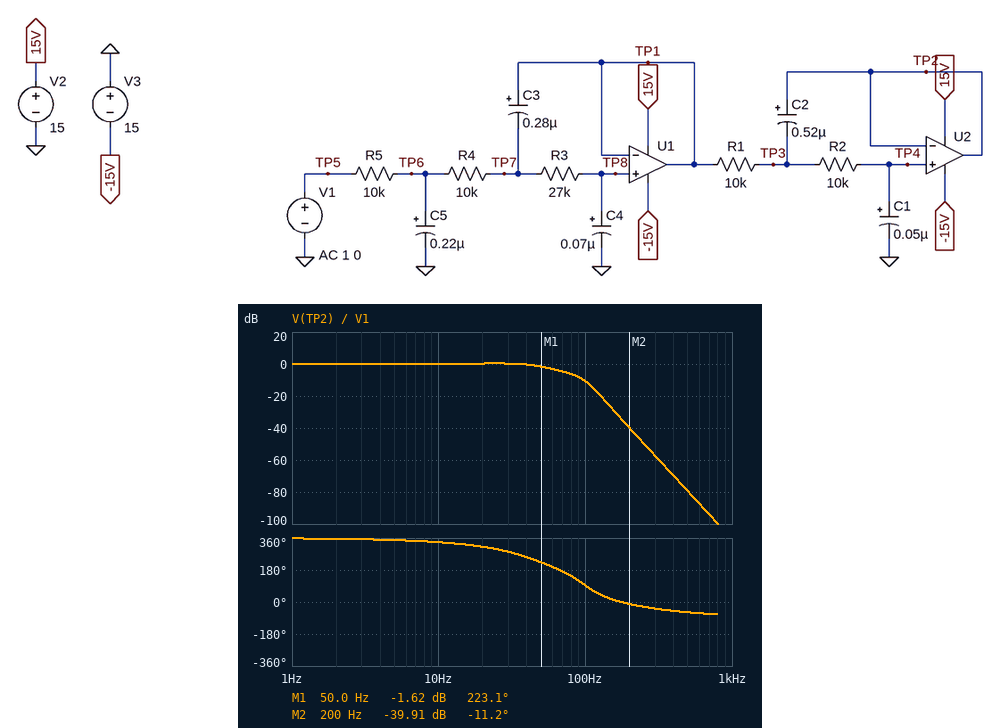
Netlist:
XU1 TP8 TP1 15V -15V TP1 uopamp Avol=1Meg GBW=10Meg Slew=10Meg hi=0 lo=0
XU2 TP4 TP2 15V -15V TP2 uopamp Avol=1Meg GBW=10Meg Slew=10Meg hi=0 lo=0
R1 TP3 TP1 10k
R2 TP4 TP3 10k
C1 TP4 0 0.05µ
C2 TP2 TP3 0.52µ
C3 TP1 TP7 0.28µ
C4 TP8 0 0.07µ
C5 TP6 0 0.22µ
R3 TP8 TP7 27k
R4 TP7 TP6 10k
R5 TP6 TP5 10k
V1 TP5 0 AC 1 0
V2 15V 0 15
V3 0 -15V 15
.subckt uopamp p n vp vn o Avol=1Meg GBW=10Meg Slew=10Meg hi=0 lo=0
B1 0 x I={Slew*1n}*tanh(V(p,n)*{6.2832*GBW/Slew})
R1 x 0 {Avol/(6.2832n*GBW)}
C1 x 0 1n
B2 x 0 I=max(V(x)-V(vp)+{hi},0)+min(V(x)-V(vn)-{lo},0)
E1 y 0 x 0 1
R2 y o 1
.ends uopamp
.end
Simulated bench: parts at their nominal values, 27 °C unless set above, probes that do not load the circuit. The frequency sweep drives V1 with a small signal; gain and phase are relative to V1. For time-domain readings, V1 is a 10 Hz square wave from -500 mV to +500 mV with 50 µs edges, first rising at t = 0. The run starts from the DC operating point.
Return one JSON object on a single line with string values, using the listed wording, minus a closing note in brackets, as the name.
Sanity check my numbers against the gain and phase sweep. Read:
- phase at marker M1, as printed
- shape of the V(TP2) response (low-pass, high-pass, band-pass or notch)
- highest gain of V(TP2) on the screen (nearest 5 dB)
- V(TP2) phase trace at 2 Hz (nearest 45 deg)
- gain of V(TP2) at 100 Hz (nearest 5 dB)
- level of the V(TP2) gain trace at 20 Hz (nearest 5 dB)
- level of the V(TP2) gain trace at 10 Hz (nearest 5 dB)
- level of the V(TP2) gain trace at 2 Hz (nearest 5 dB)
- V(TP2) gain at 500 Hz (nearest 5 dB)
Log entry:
{"phase at marker M1, as printed": "223.1 deg", "shape of the V(TP2) response": "low-pass", "highest gain of V(TP2) on the screen": "0 dB", "V(TP2) phase trace at 2 Hz": "360 deg", "gain of V(TP2) at 100 Hz": "-10 dB", "level of the V(TP2) gain trace at 20 Hz": "0 dB", "level of the V(TP2) gain trace at 10 Hz": "0 dB", "level of the V(TP2) gain trace at 2 Hz": "0 dB", "V(TP2) gain at 500 Hz": "-80 dB"}
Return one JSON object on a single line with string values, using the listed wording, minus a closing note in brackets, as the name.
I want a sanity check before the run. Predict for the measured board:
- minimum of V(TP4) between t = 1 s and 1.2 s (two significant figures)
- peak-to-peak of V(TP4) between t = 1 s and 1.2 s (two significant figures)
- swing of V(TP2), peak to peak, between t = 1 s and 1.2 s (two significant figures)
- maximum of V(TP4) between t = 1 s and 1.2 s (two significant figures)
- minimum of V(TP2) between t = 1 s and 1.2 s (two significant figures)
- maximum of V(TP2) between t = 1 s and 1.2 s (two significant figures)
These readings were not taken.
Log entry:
{"minimum of V(TP4) between t = 1 s and 1.2 s": "-580 mV", "peak-to-peak of V(TP4) between t = 1 s and 1.2 s": "1.2 V", "swing of V(TP2), peak to peak, between t = 1 s and 1.2 s": "1.2 V", "maximum of V(TP4) between t = 1 s and 1.2 s": "580 mV", "minimum of V(TP2) between t = 1 s and 1.2 s": "-580 mV", "maximum of V(TP2) between t = 1 s and 1.2 s": "580 mV"}
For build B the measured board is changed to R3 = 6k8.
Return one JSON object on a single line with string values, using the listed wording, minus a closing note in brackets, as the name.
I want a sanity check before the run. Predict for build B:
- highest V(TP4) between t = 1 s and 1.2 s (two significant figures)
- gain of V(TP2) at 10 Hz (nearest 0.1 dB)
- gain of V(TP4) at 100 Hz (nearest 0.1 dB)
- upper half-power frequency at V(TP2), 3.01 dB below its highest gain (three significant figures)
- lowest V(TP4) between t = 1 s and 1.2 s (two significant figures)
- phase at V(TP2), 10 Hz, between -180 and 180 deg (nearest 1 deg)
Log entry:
{"highest V(TP4) between t = 1 s and 1.2 s": "610 mV", "gain of V(TP2) at 10 Hz": "0 dB", "gain of V(TP4) at 100 Hz": "-2.5 dB", "upper half-power frequency at V(TP2), 3.01 dB below its highest gain": "102 Hz", "lowest V(TP4) between t = 1 s and 1.2 s": "-610 mV", "phase at V(TP2), 10 Hz, between -180 and 180 deg": "-18 deg"}
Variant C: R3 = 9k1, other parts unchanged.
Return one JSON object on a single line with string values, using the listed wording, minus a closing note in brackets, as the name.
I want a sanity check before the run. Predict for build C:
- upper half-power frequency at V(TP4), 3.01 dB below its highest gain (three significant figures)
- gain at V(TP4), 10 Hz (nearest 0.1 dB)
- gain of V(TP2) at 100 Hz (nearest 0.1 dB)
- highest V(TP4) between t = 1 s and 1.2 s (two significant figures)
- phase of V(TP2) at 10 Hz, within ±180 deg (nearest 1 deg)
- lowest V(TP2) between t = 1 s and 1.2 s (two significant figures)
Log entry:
{"upper half-power frequency at V(TP4), 3.01 dB below its highest gain": "99.0 Hz", "gain at V(TP4), 10 Hz": "0 dB", "gain of V(TP2) at 100 Hz": "-3.2 dB", "highest V(TP4) between t = 1 s and 1.2 s": "620 mV", "phase of V(TP2) at 10 Hz, within ±180 deg": "-19 deg", "lowest V(TP2) between t = 1 s and 1.2 s": "-620 mV"}
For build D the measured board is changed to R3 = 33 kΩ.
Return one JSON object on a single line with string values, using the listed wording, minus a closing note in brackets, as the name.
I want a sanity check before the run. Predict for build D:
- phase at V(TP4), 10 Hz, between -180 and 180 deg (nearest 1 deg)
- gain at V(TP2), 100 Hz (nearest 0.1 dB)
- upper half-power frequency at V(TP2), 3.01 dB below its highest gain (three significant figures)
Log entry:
{"phase at V(TP4), 10 Hz, between -180 and 180 deg": "-25 deg", "gain at V(TP2), 100 Hz": "-12.5 dB", "upper half-power frequency at V(TP2), 3.01 dB below its highest gain": "49.7 Hz"}
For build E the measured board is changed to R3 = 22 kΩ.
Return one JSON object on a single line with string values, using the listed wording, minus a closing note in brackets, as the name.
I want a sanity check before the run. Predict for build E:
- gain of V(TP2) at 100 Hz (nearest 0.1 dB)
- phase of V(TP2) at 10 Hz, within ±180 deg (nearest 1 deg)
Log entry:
{"gain of V(TP2) at 100 Hz": "-8.9 dB", "phase of V(TP2) at 10 Hz, within ±180 deg": "-22 deg"}
